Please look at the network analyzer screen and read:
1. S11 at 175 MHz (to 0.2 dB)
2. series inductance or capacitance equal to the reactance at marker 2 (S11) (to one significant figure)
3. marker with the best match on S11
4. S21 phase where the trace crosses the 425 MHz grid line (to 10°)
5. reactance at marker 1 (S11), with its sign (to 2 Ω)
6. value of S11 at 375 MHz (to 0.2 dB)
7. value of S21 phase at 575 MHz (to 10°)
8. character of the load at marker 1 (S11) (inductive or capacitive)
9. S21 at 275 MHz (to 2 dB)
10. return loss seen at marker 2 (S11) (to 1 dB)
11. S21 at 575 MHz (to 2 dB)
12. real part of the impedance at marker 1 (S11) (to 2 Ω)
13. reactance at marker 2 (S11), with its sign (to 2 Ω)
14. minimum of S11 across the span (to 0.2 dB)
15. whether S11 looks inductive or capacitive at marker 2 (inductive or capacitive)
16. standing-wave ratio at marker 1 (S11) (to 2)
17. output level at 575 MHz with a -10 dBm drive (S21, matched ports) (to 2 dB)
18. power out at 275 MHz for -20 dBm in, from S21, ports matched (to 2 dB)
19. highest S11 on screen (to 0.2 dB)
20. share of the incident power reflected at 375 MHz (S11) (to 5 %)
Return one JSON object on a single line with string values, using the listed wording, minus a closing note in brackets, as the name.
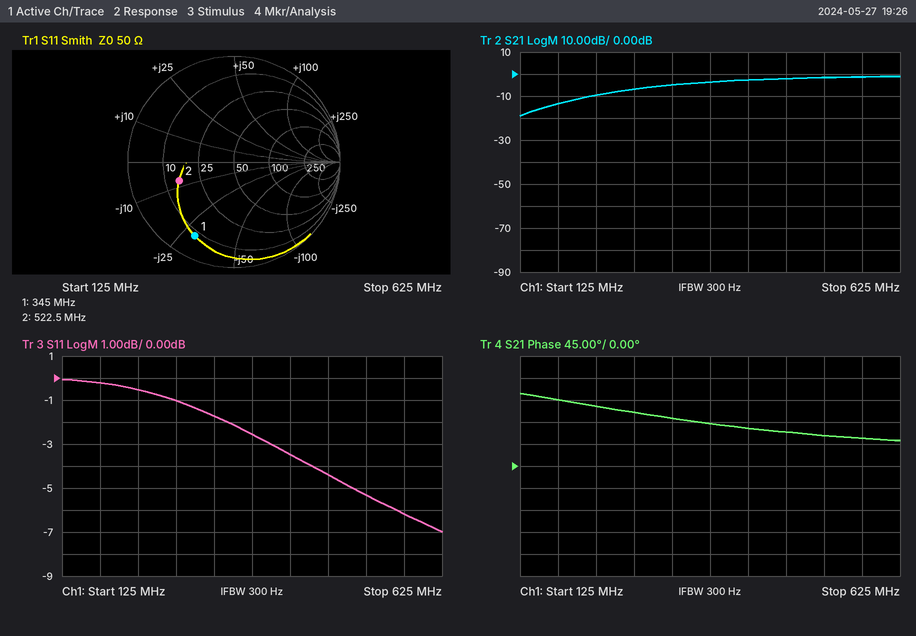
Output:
{"S11 at 175 MHz": "-0.2 dB", "series inductance or capacitance equal to the reactance at marker 2 (S11)": "40 pF", "marker with the best match on S11": "marker 2", "S21 phase where the trace crosses the 425 MHz grid line": "80°", "reactance at marker 1 (S11), with its sign": "-30 Ω", "value of S11 at 375 MHz": "-2.6 dB", "value of S21 phase at 575 MHz": "60°", "character of the load at marker 1 (S11)": "capacitive", "S21 at 275 MHz": "-6 dB", "return loss seen at marker 2 (S11)": "5 dB", "S21 at 575 MHz": "-2 dB", "real part of the impedance at marker 1 (S11)": "8 Ω", "reactance at marker 2 (S11), with its sign": "-8 Ω", "minimum of S11 across the span": "-7.0 dB", "whether S11 looks inductive or capacitive at marker 2": "capacitive", "standing-wave ratio at marker 1 (S11)": "8", "output level at 575 MHz with a -10 dBm drive (S21, matched ports)": "-12 dBm", "power out at 275 MHz for -20 dBm in, from S21, ports matched": "-26 dBm", "highest S11 on screen": "0.0 dB", "share of the incident power reflected at 375 MHz (S11)": "55 %"}
